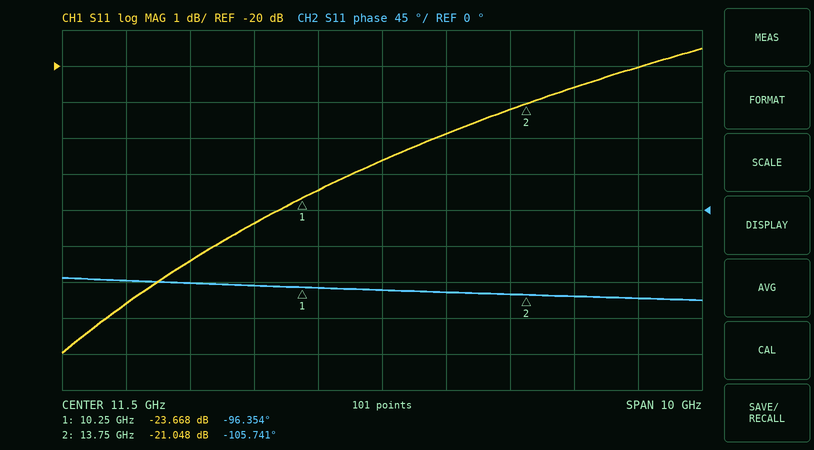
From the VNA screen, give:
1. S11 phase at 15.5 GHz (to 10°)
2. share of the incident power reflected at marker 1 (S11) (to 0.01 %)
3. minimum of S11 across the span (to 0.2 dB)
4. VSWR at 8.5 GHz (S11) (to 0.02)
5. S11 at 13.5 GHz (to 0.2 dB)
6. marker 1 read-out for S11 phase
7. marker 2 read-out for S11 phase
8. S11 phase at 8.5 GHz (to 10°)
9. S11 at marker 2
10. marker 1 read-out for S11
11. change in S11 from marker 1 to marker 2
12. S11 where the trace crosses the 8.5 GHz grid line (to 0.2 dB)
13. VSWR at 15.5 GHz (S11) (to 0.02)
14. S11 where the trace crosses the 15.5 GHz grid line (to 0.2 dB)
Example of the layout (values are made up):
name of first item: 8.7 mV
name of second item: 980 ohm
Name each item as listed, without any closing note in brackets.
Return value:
S11 phase at 15.5 GHz: -110°
share of the incident power reflected at marker 1 (S11): 0.43 %
minimum of S11 across the span: -28.0 dB
VSWR at 8.5 GHz (S11): 1.12
S11 at 13.5 GHz: -21.2 dB
marker 1 read-out for S11 phase: -96.354°
marker 2 read-out for S11 phase: -105.741°
S11 phase at 8.5 GHz: -90°
S11 at marker 2: -21.048 dB
marker 1 read-out for S11: -23.668 dB
change in S11 from marker 1 to marker 2: 2.620 dB
S11 where the trace crosses the 8.5 GHz grid line: -25.4 dB
VSWR at 15.5 GHz (S11): 1.22
S11 where the trace crosses the 15.5 GHz grid line: -20.0 dB
